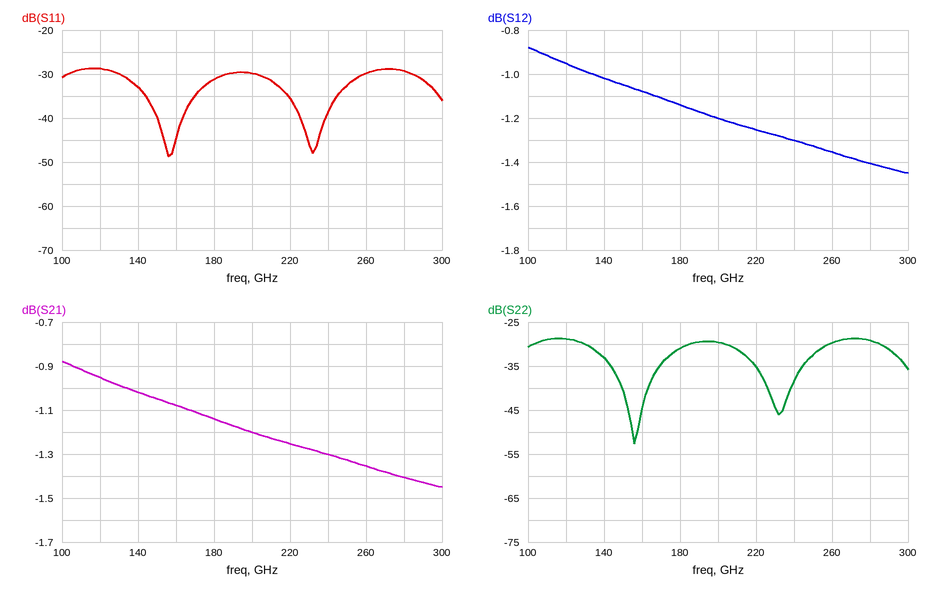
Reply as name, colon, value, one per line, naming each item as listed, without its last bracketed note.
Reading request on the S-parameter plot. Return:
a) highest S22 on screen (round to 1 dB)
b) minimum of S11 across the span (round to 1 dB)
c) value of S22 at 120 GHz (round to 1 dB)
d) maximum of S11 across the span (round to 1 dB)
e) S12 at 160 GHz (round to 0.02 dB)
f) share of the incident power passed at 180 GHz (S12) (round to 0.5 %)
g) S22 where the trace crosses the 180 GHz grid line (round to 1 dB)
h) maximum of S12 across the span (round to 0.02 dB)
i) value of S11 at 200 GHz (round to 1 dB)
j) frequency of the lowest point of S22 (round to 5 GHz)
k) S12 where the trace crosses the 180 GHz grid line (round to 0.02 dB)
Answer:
highest S22 on screen: -29 dB
minimum of S11 across the span: -49 dB
value of S22 at 120 GHz: -29 dB
maximum of S11 across the span: -29 dB
S12 at 160 GHz: -1.08 dB
share of the incident power passed at 180 GHz (S12): 77.0 %
S22 where the trace crosses the 180 GHz grid line: -31 dB
maximum of S12 across the span: -0.88 dB
value of S11 at 200 GHz: -30 dB
frequency of the lowest point of S22: 155 GHz
S12 where the trace crosses the 180 GHz grid line: -1.14 dB
